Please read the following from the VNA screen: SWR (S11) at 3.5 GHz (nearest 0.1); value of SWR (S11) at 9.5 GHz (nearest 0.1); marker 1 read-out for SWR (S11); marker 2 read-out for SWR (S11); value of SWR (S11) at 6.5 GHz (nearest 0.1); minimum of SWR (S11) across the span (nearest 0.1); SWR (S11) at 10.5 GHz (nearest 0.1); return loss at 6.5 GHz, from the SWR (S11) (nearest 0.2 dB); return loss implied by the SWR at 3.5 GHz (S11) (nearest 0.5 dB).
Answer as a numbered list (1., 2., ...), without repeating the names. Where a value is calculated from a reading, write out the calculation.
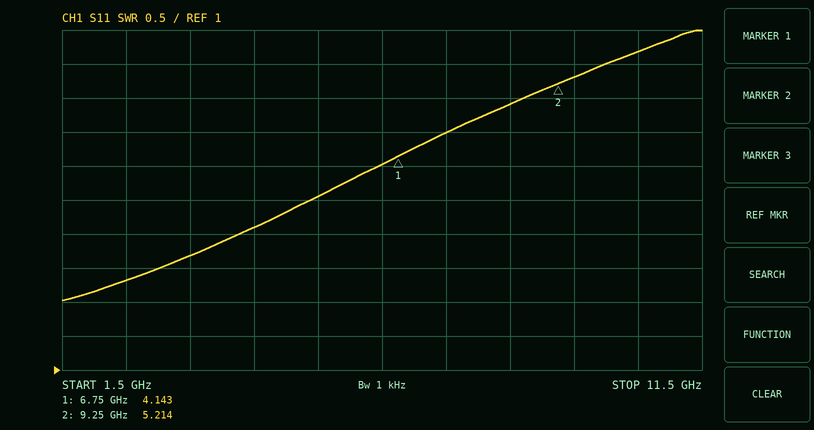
1. 2.7
2. 5.3
3. 4.143
4. 5.214
5. 4.0
6. 2.0
7. 5.7
8. −20 log10((4 − 1)/(4 + 1)) ≈ 4.4 dB
9. −20 log10((2.7 − 1)/(2.7 + 1)) ≈ 6.76 dB, so 7.0 dB to the nearest 0.5 dB
